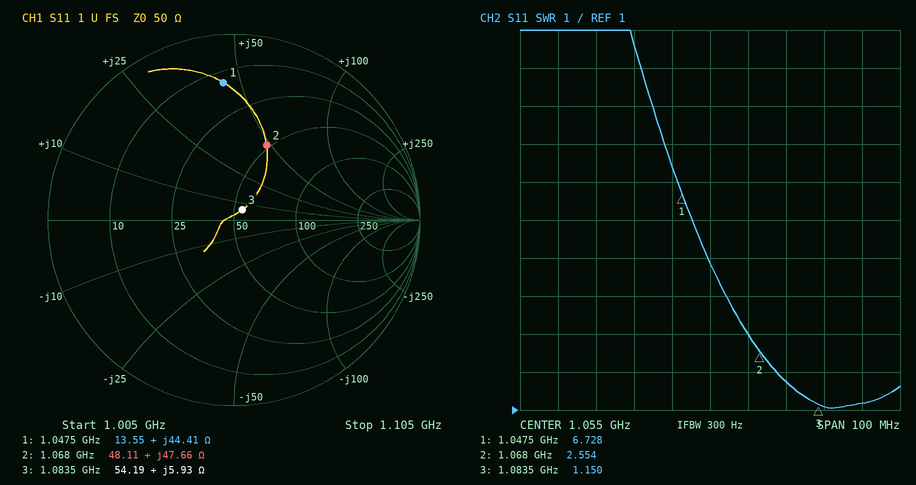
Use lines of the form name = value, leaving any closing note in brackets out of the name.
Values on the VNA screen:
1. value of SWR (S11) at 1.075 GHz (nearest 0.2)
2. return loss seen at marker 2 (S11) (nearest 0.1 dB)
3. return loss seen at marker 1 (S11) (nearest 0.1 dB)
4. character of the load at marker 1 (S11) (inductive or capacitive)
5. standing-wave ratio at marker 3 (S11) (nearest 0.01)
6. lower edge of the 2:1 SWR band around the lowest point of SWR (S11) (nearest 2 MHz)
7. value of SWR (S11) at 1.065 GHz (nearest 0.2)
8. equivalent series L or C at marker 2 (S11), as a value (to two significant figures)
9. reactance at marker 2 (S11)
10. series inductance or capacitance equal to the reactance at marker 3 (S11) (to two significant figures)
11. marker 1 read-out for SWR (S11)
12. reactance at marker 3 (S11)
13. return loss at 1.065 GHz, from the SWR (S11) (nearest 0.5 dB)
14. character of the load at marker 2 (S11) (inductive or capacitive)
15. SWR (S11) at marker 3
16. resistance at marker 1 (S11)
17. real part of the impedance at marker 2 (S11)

value of SWR (S11) at 1.075 GHz = 1.8
return loss seen at marker 2 (S11) = 7.2 dB
return loss seen at marker 1 (S11) = 2.6 dB
character of the load at marker 1 (S11) = inductive
standing-wave ratio at marker 3 (S11) = 1.15
lower edge of the 2:1 SWR band around the lowest point of SWR (S11) = 1.072 GHz
value of SWR (S11) at 1.065 GHz = 3.0
equivalent series L or C at marker 2 (S11), as a value = 7.1 nH
reactance at marker 2 = +47.66 Ω
series inductance or capacitance equal to the reactance at marker 3 (S11) = 870 pH
marker 1 read-out for SWR = 6.728
reactance at marker 3 = +5.93 Ω
return loss at 1.065 GHz, from the SWR (S11) = 6.0 dB
character of the load at marker 2 (S11) = inductive
SWR (S11) at marker 3 = 1.150
resistance at marker 1 = 13.55 Ω
real part of the impedance at marker 2 = 48.11 Ω
